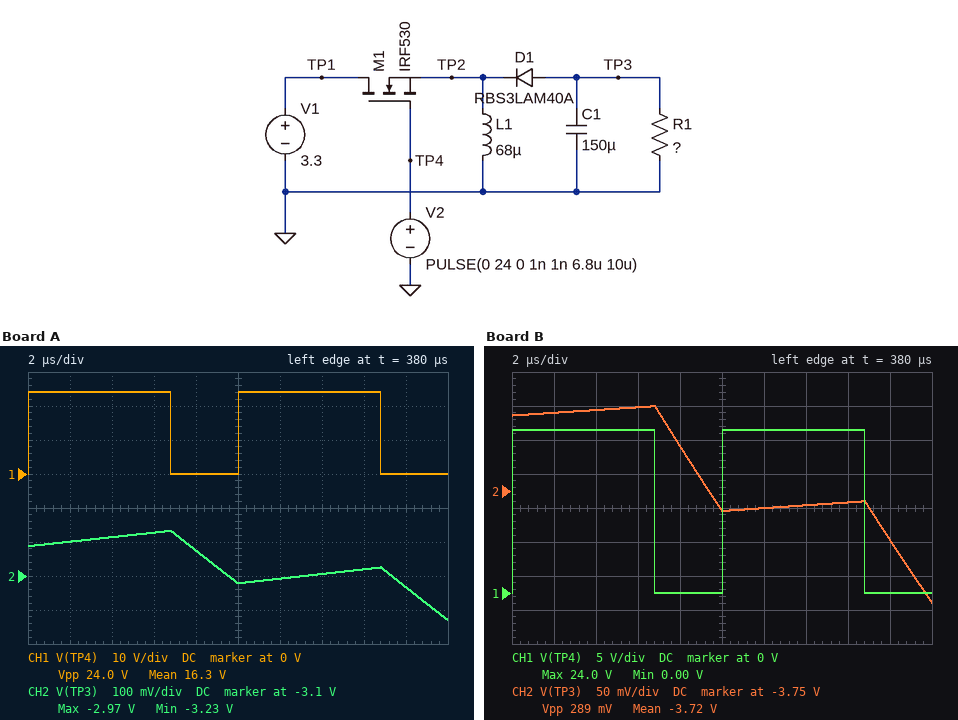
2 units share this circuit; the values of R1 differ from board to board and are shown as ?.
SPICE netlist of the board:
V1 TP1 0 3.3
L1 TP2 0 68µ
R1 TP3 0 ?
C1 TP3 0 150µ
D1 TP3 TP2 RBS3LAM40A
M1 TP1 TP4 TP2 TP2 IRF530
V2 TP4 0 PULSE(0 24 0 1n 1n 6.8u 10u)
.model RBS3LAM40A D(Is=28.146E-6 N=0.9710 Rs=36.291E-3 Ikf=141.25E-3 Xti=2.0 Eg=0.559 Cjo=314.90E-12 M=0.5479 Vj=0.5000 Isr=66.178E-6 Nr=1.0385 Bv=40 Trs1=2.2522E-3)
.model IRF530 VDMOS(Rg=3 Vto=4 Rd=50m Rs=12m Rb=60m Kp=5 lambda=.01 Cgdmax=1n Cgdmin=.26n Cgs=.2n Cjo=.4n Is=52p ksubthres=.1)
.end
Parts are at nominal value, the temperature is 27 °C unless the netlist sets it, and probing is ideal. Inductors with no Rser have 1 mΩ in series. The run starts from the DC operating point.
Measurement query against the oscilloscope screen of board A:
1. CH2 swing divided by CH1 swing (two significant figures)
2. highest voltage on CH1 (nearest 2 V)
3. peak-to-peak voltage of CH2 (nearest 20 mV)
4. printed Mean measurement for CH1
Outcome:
0.011
24 V
260 mV
16.3 V
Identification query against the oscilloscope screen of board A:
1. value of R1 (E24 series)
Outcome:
3 Ω
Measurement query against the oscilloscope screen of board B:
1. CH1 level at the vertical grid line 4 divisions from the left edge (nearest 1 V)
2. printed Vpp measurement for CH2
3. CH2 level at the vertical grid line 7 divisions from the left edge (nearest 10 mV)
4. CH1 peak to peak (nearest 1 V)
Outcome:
0 V
289 mV
-3.77 V
24 V
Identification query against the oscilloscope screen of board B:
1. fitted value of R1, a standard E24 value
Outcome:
12 Ω
